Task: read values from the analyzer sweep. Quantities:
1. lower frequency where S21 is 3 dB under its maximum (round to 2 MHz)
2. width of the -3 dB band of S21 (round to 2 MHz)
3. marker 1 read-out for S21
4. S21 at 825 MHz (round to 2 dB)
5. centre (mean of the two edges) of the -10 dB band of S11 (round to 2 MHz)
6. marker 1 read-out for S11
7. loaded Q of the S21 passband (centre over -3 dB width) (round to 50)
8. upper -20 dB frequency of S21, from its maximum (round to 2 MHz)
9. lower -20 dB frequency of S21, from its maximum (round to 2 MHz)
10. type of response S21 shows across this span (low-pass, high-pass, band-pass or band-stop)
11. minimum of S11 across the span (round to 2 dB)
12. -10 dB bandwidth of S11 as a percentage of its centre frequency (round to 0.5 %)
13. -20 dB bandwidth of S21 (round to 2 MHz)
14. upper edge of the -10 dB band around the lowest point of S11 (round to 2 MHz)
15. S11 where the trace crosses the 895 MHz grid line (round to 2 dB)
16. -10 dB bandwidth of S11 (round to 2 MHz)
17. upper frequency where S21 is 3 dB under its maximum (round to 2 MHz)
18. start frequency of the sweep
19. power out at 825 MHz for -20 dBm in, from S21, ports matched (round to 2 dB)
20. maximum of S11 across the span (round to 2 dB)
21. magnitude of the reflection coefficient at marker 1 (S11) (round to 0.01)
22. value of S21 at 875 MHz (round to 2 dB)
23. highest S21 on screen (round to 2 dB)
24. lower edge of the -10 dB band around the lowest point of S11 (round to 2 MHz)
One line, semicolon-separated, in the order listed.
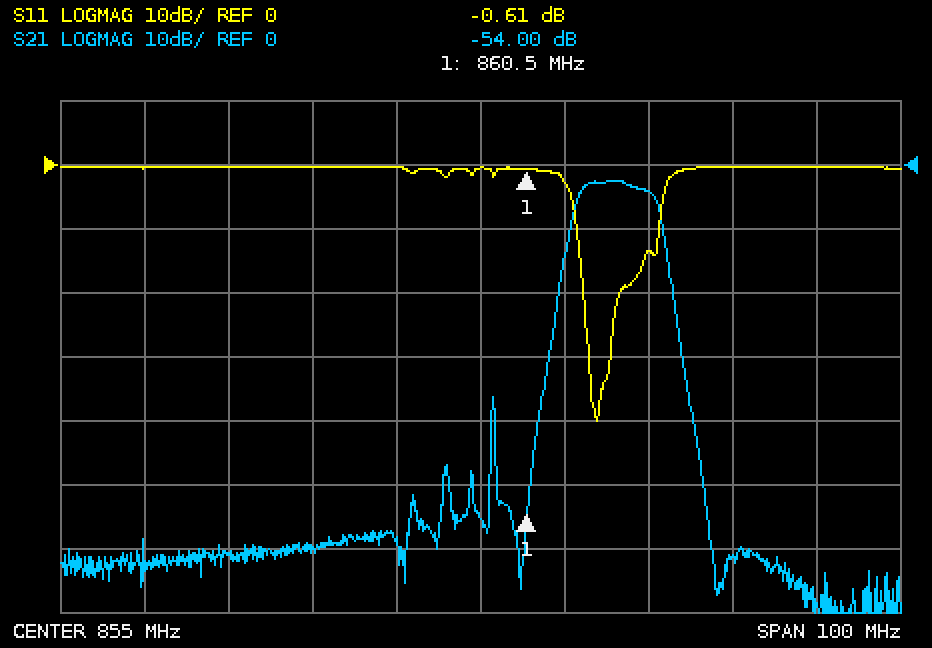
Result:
866 MHz; 10 MHz; -54.00 dB; -60 dB; 872 MHz; -0.61 dB; 100; 878 MHz; 864 MHz; band-pass; -40 dB; 1.0 %; 14 MHz; 876 MHz; 0 dB; 10 MHz; 876 MHz; 805 MHz; -80 dBm; 0 dB; 0.93; -4 dB; -2 dB; 866 MHz
